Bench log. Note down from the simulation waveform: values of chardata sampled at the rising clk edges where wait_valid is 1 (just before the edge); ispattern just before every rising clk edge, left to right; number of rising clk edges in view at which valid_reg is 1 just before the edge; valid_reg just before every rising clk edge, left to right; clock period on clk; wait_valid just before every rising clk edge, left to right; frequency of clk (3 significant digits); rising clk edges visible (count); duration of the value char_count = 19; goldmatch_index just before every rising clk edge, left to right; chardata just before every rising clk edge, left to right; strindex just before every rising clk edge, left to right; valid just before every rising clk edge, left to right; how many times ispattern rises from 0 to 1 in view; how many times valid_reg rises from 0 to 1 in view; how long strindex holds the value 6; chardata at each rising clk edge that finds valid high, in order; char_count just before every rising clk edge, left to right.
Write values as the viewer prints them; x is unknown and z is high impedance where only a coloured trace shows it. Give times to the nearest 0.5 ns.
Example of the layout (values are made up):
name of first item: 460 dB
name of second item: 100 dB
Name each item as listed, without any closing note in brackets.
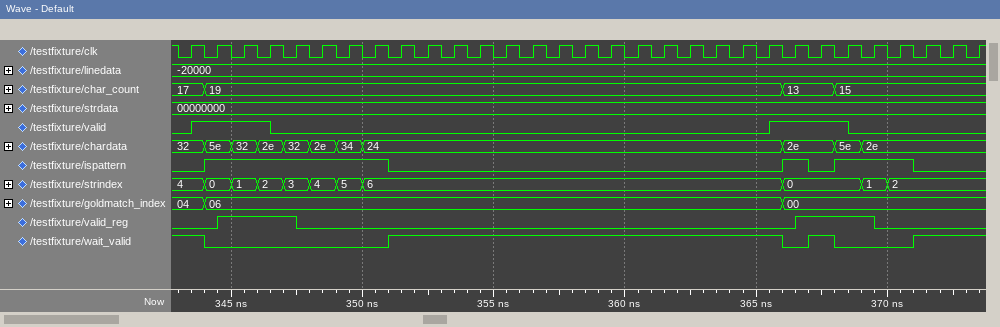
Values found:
values of chardata sampled at the rising clk edges where wait_valid is 1: 32, 24, 24, 24, 24, 24, 24, 24, 24, 24, 24, 24, 24, 24, 24, 24, 2e, 2e, 2e, 2e
ispattern just before every rising clk edge, left to right: 0 1 1 1 1 1 1 1 0 0 0 0 0 0 0 0 0 0 0 0 0 0 0 1 0 1 1 1 0 0 0
number of rising clk edges in view at which valid_reg is 1 just before the edge: 6
valid_reg just before every rising clk edge, left to right: 0 0 1 1 1 0 0 0 0 0 0 0 0 0 0 0 0 0 0 0 0 0 0 0 1 1 1 0 0 0 0
clock period on clk: 1 ns
wait_valid just before every rising clk edge, left to right: 1 0 0 0 0 0 0 0 1 1 1 1 1 1 1 1 1 1 1 1 1 1 1 0 1 0 0 0 1 1 1
frequency of clk: 1.00 GHz
rising clk edges visible: 31
duration of the value char_count = 19: 22 ns
goldmatch_index just before every rising clk edge, left to right: 04, 06, 06, 06, 06, 06, 06, 06, 06, 06, 06, 06, 06, 06, 06, 06, 06, 06, 06, 06, 06, 06, 06, 00, 00, 00, 00, 00, 00, 00, 00
chardata just before every rising clk edge, left to right: 32, 5e, 32, 2e, 32, 2e, 34, 24, 24, 24, 24, 24, 24, 24, 24, 24, 24, 24, 24, 24, 24, 24, 24, 2e, 2e, 5e, 2e, 2e, 2e, 2e, 2e
strindex just before every rising clk edge, left to right: 4, 0, 1, 2, 3, 4, 5, 6, 6, 6, 6, 6, 6, 6, 6, 6, 6, 6, 6, 6, 6, 6, 6, 0, 0, 0, 1, 2, 2, 2, 2
valid just before every rising clk edge, left to right: 0 1 1 1 0 0 0 0 0 0 0 0 0 0 0 0 0 0 0 0 0 0 0 1 1 1 0 0 0 0 0
how many times ispattern rises from 0 to 1 in view: 3
how many times valid_reg rises from 0 to 1 in view: 2
how long strindex holds the value 6: 16 ns
chardata at each rising clk edge that finds valid high, in order: 5e, 32, 2e, 2e, 2e, 5e
char_count just before every rising clk edge, left to right: 17, 19, 19, 19, 19, 19, 19, 19, 19, 19, 19, 19, 19, 19, 19, 19, 19, 19, 19, 19, 19, 19, 19, 13, 13, 15, 15, 15, 15, 15, 15
